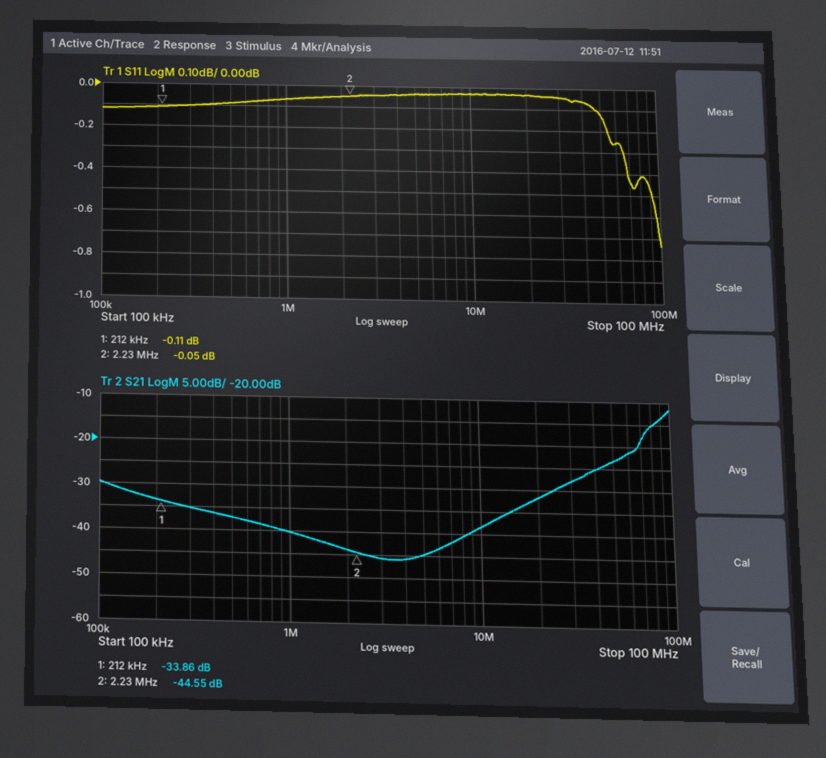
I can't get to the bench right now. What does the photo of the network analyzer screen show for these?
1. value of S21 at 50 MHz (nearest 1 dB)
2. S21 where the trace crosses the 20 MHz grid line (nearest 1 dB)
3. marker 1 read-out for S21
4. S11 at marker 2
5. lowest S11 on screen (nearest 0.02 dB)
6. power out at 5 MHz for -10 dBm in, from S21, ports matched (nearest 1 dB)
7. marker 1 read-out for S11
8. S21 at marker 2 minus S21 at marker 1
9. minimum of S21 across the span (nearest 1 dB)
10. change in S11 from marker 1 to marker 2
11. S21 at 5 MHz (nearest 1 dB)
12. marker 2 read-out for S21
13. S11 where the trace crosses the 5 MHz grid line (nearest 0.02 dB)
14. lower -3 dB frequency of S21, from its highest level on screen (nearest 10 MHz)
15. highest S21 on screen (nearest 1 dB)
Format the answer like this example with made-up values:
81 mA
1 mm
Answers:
-23 dB
-32 dB
-33.86 dB
-0.05 dB
-0.74 dB
-55 dBm
-0.11 dB
-10.69 dB
-46 dB
0.06 dB
-45 dB
-44.55 dB
-0.04 dB
80 MHz
-12 dB
